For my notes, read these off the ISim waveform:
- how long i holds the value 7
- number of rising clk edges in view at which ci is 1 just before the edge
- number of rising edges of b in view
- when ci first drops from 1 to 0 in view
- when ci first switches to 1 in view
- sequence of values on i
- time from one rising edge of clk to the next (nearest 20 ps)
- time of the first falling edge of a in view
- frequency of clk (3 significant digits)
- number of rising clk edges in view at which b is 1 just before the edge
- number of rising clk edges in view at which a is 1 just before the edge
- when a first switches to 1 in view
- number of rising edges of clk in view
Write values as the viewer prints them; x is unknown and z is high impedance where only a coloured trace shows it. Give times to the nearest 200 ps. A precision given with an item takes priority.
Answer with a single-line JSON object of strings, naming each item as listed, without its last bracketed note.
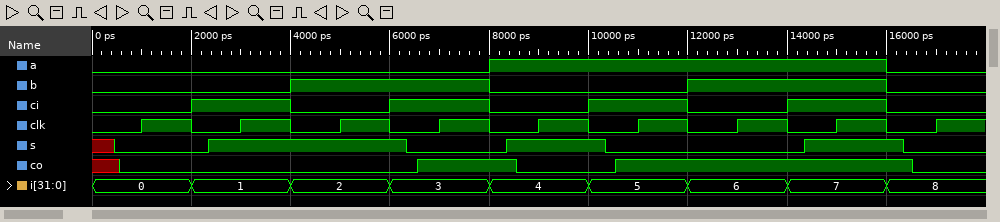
{"how long i holds the value 7": "2000 ps", "number of rising clk edges in view at which ci is 1 just before the edge": "4", "number of rising edges of b in view": "2", "when ci first drops from 1 to 0 in view": "4000 ps", "when ci first switches to 1 in view": "2000 ps", "sequence of values on i": "0, 1, 2, 3, 4, 5, 6, 7, 8", "time from one rising edge of clk to the next": "2000 ps", "time of the first falling edge of a in view": "16000 ps", "frequency of clk": "500 MHz", "number of rising clk edges in view at which b is 1 just before the edge": "4", "number of rising clk edges in view at which a is 1 just before the edge": "4", "when a first switches to 1 in view": "8000 ps", "number of rising edges of clk in view": "9"}
